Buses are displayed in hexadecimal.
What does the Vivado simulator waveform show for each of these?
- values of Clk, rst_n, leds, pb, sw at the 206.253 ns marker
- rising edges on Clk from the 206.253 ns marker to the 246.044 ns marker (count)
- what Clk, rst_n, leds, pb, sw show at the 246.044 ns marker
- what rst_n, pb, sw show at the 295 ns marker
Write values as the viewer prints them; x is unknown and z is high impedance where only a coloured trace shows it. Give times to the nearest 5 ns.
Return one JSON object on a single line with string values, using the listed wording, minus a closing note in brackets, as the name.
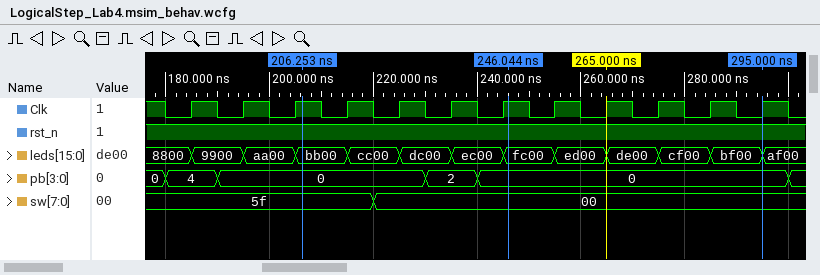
{"values of Clk, rst_n, leds, pb, sw at the 206.253 ns marker": "Clk=1, rst_n=1, leds=bb00, pb=0, sw=5f", "rising edges on Clk from the 206.253 ns marker to the 246.044 ns marker": "4", "what Clk, rst_n, leds, pb, sw show at the 246.044 ns marker": "Clk=1, rst_n=1, leds=fc00, pb=0, sw=00", "what rst_n, pb, sw show at the 295 ns marker": "rst_n=1, pb=0, sw=00"}
